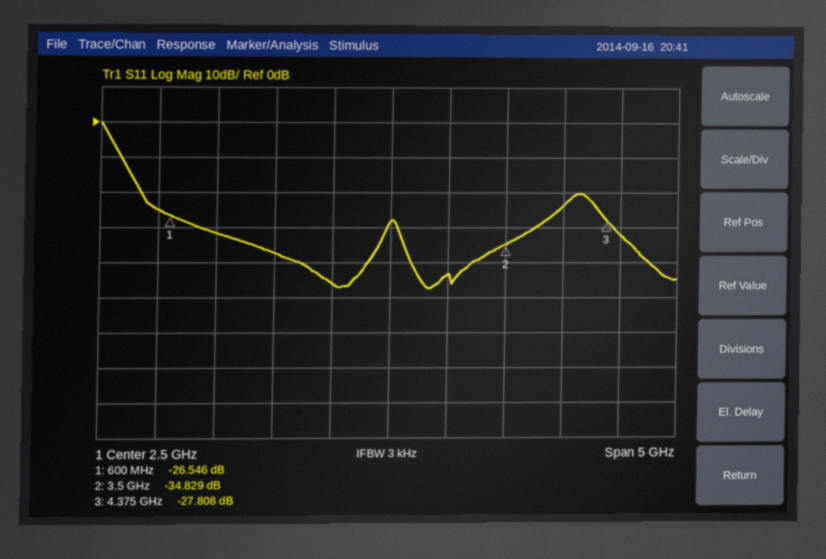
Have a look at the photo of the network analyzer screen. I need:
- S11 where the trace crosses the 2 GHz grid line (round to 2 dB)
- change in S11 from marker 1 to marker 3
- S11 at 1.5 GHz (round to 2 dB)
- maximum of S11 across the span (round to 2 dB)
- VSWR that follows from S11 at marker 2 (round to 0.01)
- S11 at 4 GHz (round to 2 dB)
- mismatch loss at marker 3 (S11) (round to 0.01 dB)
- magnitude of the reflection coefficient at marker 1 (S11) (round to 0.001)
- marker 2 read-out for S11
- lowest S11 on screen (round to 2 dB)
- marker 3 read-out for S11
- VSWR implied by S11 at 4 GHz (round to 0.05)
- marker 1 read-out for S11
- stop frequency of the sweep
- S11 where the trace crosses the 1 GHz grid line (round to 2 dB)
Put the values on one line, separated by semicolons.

-46 dB; -1.262 dB; -38 dB; 0 dB; 1.04; -24 dB; 0.01 dB; 0.047; -34.829 dB; -48 dB; -27.808 dB; 1.15; -26.546 dB; 5 GHz; -32 dB
